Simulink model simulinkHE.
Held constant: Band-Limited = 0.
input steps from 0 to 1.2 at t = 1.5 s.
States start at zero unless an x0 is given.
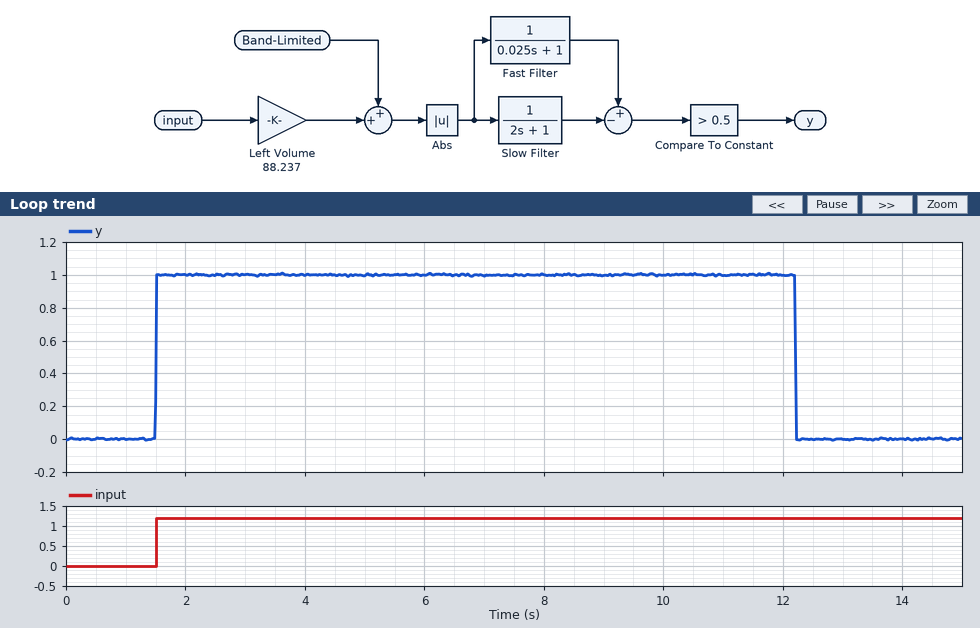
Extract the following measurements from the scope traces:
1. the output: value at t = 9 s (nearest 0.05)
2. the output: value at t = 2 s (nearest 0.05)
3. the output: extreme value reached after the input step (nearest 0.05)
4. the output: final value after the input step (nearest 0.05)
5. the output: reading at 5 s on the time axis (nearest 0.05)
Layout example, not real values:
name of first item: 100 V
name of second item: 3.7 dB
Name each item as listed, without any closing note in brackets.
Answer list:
the output: value at t = 9 s: 1.00
the output: value at t = 2 s: 1.00
the output: extreme value reached after the input step: 1.00
the output: final value after the input step: 0.00
the output: reading at 5 s on the time axis: 1.00
